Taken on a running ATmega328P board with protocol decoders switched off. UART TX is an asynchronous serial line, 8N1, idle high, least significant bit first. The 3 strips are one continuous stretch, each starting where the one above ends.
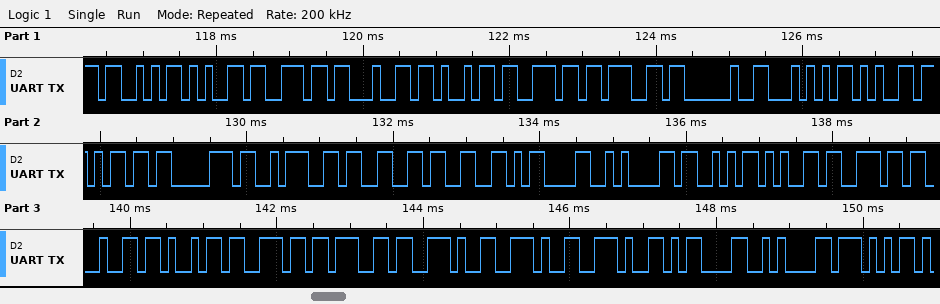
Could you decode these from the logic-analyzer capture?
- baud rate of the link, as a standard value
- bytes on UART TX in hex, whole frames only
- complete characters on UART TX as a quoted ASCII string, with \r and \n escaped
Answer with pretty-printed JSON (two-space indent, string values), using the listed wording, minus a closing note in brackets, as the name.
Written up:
{
  "baud rate of the link, as a standard value": "9600 baud",
  "bytes on UART TX in hex, whole frames only": "0x53 0x65 0x6E 0x64 0x69 0x6E 0x67 0x20 0x54 0x65 0x6D 0x70 0x3A 0x33 0x33 0x0D 0x0A 0x53 0x65 0x6E 0x64 0x69 0x6E 0x67 0x2E 0x2E 0x2E 0x0D 0x0A 0x57",
  "complete characters on UART TX as a quoted ASCII string, with \\r and \\n escaped": "\"Sending Temp:33\\r\\nSending...\\r\\nW\""
}
